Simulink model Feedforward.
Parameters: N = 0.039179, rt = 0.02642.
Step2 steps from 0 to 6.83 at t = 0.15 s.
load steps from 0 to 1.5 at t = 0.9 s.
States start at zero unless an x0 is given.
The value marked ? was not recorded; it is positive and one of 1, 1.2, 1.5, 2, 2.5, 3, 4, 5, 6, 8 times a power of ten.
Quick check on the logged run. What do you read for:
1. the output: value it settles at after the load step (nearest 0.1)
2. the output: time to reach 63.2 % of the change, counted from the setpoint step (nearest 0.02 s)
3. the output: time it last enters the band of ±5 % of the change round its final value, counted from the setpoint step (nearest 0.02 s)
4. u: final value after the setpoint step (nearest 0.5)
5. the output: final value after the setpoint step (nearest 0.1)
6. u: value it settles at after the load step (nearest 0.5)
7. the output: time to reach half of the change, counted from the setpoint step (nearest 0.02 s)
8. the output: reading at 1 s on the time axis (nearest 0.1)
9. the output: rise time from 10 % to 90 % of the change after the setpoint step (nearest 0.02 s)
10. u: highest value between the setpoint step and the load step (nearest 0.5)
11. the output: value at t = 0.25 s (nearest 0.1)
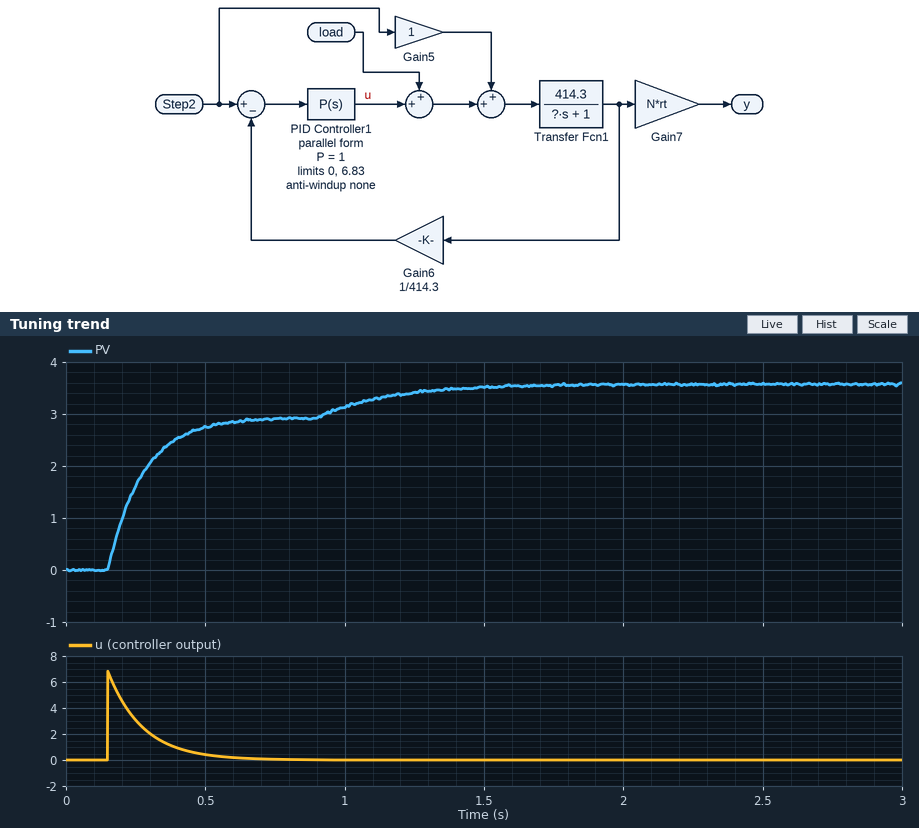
3.6
0.12 s
0.38 s
0.0
2.9
0.0
0.08 s
3.1
0.28 s
7.0
1.6
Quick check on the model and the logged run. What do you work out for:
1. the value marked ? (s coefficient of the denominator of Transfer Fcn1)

0.25
